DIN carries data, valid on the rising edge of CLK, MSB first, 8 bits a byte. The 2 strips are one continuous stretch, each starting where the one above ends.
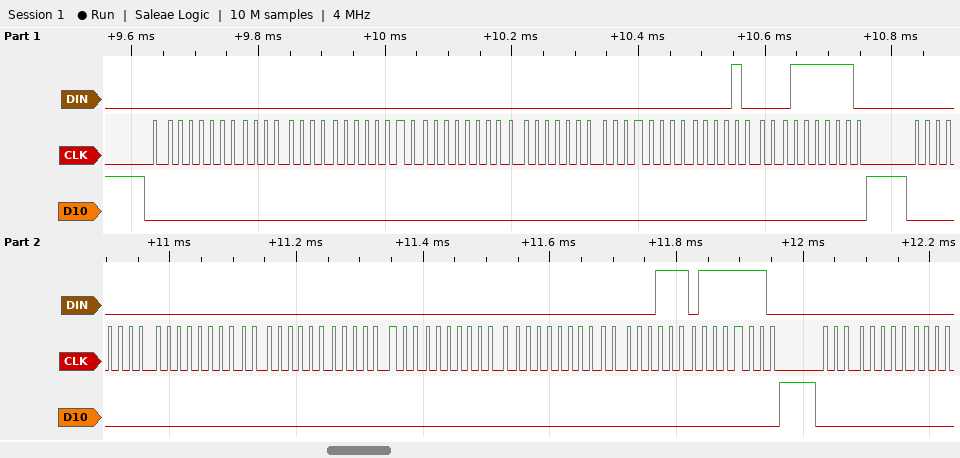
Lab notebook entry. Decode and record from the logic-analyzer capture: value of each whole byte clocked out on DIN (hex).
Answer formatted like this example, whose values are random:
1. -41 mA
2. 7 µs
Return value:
1. 00 00 00 00 00 00 08 7E 00 00 00 00 00 00 07 7E 00
